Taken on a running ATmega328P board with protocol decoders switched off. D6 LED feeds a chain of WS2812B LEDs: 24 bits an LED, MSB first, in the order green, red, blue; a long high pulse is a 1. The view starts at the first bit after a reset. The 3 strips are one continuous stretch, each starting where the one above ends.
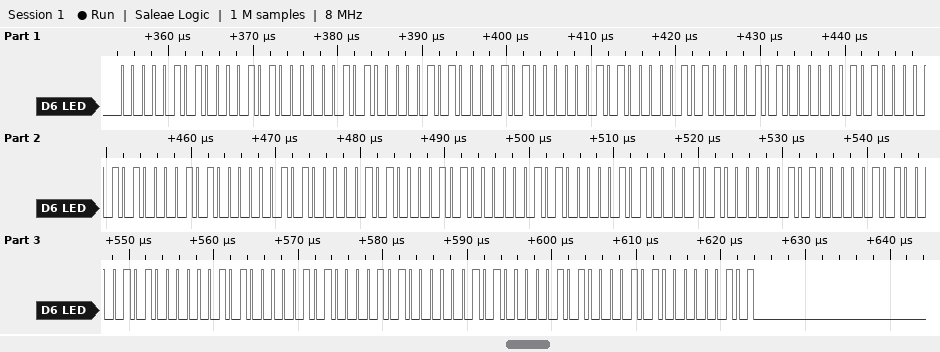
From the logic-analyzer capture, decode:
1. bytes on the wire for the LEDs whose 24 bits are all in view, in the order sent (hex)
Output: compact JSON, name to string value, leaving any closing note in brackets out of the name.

{"bytes on the wire for the LEDs whose 24 bits are all in view, in the order sent": "05 0A 05 05 0A 05 05 0A 05 05 0A 05 05 0A 05 05 0A 05 05 0A 05 05 0A 05 05 0A 05"}
